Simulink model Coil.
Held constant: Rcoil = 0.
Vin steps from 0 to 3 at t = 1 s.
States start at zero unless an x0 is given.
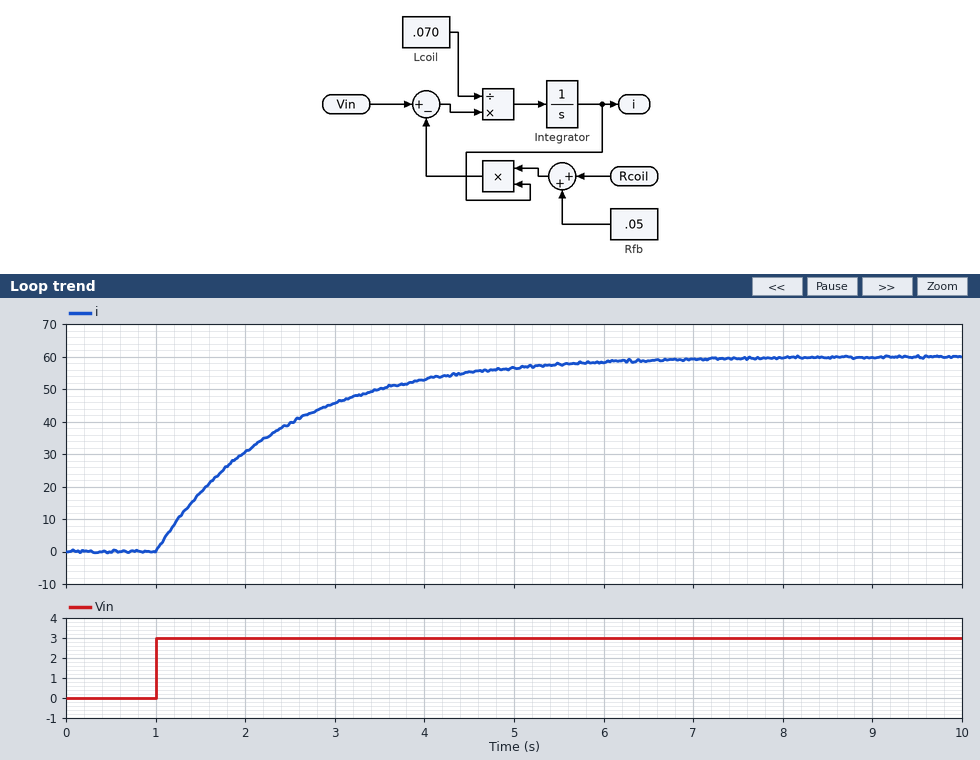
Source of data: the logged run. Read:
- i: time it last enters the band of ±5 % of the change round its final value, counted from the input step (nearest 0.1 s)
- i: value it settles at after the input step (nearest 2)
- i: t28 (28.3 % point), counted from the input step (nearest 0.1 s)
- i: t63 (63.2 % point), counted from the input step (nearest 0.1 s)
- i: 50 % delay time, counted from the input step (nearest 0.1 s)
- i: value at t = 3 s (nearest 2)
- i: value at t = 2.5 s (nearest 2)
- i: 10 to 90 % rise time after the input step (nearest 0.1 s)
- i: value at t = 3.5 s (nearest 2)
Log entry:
4.2 s
60
0.5 s
1.4 s
1.0 s
46
40
3.1 s
50
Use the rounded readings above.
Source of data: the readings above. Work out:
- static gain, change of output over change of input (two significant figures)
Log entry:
20
